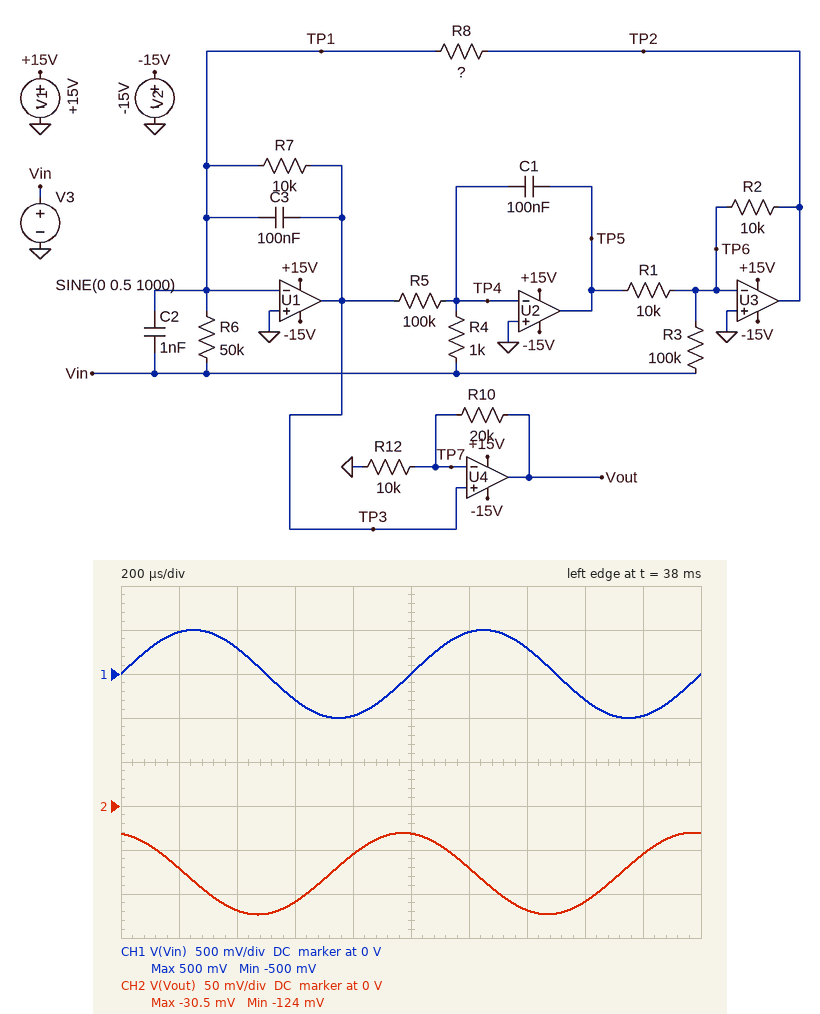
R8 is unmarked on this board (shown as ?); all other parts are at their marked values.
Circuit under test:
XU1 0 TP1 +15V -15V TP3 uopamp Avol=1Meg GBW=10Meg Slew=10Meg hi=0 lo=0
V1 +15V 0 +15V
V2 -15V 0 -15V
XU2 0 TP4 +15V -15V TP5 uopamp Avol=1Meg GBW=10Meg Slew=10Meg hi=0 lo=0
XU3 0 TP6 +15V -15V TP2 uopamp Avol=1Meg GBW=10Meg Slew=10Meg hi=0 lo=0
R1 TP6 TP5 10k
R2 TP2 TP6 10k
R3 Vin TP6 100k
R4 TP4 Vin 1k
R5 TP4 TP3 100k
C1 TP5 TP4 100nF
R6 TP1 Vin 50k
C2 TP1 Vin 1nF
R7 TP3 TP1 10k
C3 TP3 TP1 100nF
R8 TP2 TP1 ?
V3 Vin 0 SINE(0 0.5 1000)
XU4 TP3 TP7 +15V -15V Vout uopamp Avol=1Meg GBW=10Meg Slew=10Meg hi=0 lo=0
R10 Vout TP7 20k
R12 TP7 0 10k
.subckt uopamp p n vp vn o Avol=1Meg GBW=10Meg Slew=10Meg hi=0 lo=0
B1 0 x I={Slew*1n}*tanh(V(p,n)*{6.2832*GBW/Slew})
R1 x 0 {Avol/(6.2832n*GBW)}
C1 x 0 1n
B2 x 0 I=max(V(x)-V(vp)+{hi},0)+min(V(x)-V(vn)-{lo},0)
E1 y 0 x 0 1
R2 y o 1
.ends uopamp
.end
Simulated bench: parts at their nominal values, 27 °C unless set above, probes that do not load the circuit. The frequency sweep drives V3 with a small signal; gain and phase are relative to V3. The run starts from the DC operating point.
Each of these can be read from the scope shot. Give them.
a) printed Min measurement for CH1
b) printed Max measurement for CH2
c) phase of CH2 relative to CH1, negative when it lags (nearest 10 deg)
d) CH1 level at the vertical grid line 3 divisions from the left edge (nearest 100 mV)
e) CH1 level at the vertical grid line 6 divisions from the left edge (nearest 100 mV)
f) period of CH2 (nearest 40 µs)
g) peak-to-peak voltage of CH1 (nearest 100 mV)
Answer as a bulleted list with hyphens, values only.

- -500 mV
- -30.5 mV
- 100 deg
- -300 mV
- 500 mV
- 1.00 ms
- 1.0 V
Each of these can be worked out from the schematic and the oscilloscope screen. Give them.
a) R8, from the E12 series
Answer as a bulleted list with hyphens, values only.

- 270 kΩ
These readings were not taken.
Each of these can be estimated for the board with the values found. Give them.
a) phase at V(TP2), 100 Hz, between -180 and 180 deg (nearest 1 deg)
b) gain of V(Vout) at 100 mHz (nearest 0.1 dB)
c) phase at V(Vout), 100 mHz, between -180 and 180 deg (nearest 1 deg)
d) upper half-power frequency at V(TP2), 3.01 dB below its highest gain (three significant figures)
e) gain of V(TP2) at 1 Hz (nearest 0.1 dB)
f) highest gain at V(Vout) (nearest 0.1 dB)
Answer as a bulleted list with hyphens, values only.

- -90 deg
- 49.4 dB
- 170 deg
- 593 mHz
- 62.7 dB
- 49.5 dB
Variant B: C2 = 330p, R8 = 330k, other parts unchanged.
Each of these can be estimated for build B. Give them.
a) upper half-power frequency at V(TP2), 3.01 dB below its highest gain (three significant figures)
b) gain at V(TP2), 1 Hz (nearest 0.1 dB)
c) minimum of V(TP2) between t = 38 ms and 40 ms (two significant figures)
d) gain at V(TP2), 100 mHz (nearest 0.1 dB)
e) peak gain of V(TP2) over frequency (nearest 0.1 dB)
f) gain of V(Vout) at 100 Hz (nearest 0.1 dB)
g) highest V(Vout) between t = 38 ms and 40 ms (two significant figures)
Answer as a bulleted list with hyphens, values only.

- 485 mHz
- 63.1 dB
- -91 mV
- 70.1 dB
- 70.3 dB
- 2.4 dB
- -17 mV
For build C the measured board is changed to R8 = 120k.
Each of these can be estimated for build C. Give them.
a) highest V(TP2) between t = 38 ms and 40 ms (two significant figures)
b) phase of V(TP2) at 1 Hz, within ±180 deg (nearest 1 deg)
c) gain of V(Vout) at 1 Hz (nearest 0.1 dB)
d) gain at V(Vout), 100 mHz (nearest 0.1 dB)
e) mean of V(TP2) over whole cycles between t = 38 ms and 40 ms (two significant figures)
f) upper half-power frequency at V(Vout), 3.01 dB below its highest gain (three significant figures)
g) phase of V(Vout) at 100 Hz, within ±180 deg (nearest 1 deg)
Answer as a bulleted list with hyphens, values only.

- 1.4 V
- -37 deg
- 47.6 dB
- 49.5 dB
- 580 mV
- 1.34 Hz
- 67 deg
